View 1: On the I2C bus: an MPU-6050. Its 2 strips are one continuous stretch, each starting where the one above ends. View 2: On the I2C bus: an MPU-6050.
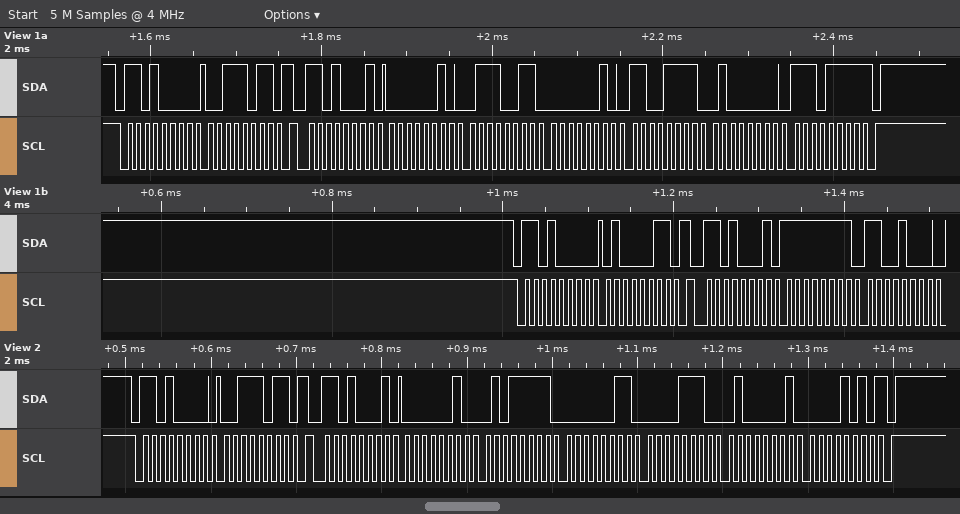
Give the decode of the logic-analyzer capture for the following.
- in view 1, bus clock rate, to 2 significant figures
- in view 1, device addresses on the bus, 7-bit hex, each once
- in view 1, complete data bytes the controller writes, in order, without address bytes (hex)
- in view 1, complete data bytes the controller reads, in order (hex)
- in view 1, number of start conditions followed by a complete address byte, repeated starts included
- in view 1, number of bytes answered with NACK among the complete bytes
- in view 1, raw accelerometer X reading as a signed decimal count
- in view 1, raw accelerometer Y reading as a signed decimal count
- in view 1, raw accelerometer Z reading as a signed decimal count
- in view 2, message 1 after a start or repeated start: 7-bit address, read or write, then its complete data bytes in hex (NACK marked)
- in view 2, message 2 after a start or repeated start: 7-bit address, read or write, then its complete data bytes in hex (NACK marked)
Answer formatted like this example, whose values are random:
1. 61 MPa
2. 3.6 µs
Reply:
1. 100 kHz
2. 0x68
3. 3B 43
4. 02 73 02 CF 40 EF FF C8
5. 4
6. 1
7. 627
8. 719
9. 16623
10. 0x68 write: 3B
11. 0x68 read: 02 5F 03 0E 41 0A NACK
